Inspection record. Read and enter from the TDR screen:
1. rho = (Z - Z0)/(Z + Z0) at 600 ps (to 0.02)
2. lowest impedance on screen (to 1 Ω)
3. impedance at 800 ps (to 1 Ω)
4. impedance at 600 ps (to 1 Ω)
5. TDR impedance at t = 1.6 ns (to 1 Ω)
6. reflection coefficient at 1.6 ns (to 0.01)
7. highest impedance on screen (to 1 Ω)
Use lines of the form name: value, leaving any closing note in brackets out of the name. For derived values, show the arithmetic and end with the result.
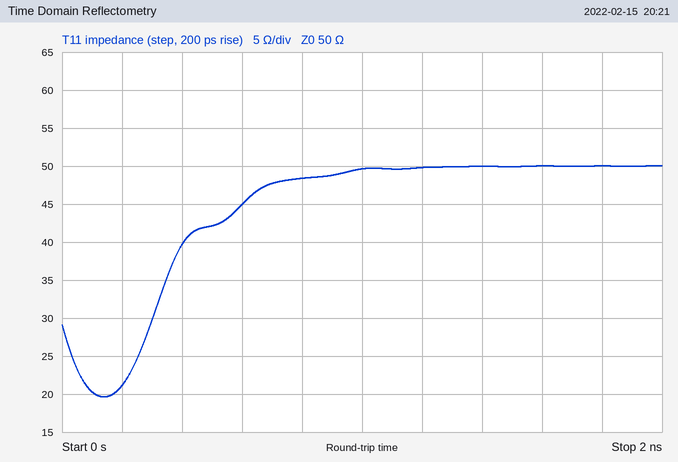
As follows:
rho = (Z - Z0)/(Z + Z0) at 600 ps: (45 − 50)/(45 + 50) ≈ -0.0526, so -0.06 to the nearest 0.02
lowest impedance on screen: 20 Ω
impedance at 800 ps: 48 Ω
impedance at 600 ps: 45 Ω
TDR impedance at t = 1.6 ns: 50 Ω
reflection coefficient at 1.6 ns: (50 − 50)/(50 + 50) ≈ 0.00
highest impedance on screen: 50 Ω
